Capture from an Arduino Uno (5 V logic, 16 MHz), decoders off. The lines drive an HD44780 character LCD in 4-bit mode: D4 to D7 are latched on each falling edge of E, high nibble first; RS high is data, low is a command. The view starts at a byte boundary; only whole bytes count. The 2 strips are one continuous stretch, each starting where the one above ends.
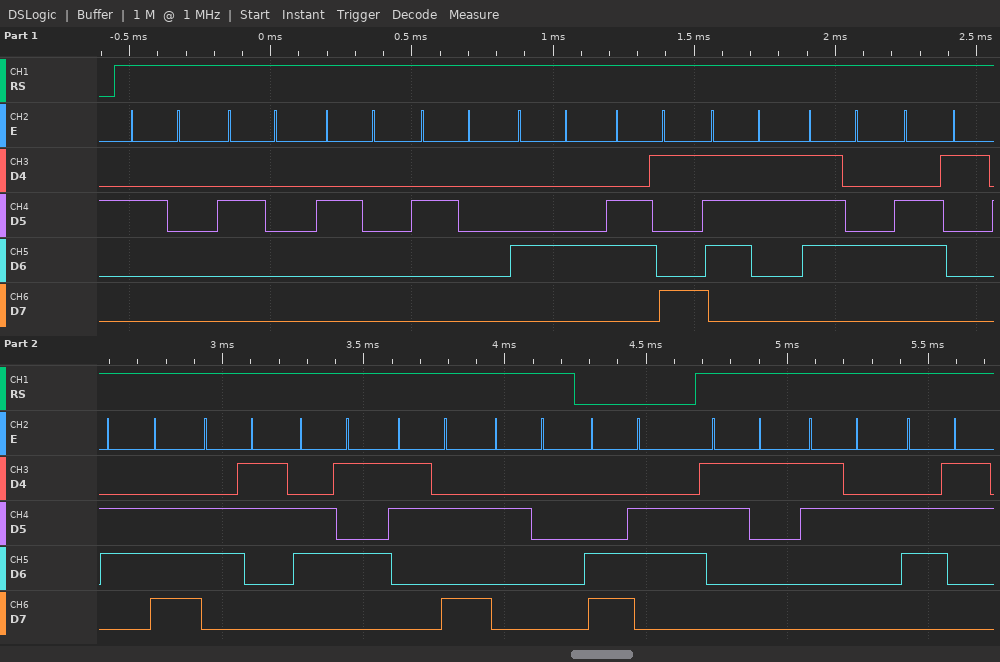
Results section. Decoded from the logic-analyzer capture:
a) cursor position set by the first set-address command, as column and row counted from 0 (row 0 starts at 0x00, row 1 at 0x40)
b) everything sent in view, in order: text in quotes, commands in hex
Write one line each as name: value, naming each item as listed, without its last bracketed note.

cursor position set by the first set-address command, as column and row counted from 0: column 6, row 1
everything sent in view, in order: text in quotes, commands in hex: "    Distance: " 0xC6 "12c"
